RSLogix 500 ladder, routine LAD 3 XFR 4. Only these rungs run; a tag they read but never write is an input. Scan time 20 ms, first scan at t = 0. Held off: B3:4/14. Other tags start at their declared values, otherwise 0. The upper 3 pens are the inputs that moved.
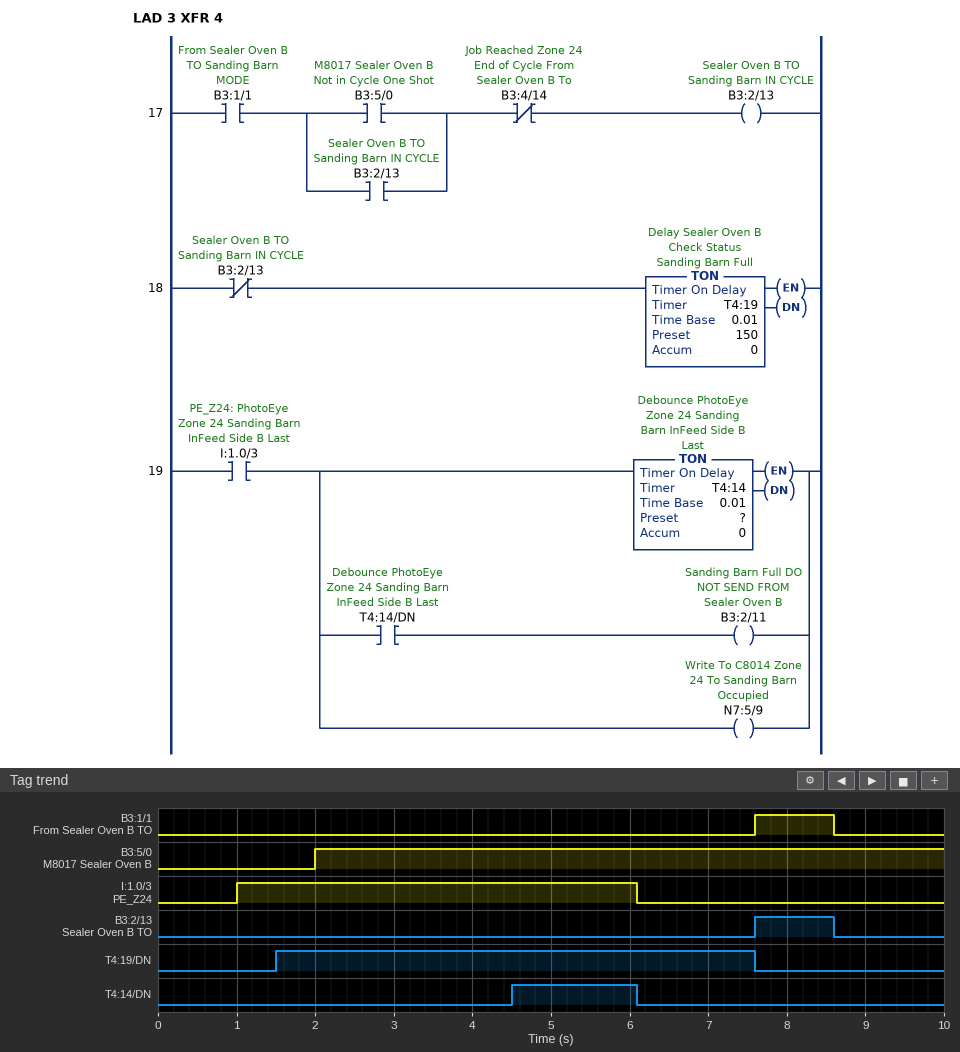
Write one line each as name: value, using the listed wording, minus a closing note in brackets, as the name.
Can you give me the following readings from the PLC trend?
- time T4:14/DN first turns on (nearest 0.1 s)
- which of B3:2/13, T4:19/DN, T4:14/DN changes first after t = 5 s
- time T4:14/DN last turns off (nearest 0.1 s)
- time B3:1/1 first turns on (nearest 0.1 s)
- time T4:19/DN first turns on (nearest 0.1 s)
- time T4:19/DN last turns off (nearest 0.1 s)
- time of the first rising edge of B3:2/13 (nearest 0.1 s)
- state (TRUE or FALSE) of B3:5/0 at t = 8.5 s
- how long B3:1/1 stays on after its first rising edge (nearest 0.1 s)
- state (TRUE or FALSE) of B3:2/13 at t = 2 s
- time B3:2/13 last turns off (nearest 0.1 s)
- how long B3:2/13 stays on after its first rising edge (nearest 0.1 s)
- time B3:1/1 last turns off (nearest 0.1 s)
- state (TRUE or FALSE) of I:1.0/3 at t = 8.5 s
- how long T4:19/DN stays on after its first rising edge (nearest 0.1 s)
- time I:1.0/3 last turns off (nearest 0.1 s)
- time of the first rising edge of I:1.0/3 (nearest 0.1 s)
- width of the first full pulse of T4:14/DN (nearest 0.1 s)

time T4:14/DN first turns on: 4.5 s
which of B3:2/13, T4:19/DN, T4:14/DN changes first after t = 5 s: T4:14/DN
time T4:14/DN last turns off: 6.1 s
time B3:1/1 first turns on: 7.6 s
time T4:19/DN first turns on: 1.5 s
time T4:19/DN last turns off: 7.6 s
time of the first rising edge of B3:2/13: 7.6 s
state (TRUE or FALSE) of B3:5/0 at t = 8.5 s: TRUE
how long B3:1/1 stays on after its first rising edge: 1.0 s
state (TRUE or FALSE) of B3:2/13 at t = 2 s: FALSE
time B3:2/13 last turns off: 8.6 s
how long B3:2/13 stays on after its first rising edge: 1.0 s
time B3:1/1 last turns off: 8.6 s
state (TRUE or FALSE) of I:1.0/3 at t = 8.5 s: FALSE
how long T4:19/DN stays on after its first rising edge: 6.1 s
time I:1.0/3 last turns off: 6.1 s
time of the first rising edge of I:1.0/3: 1.0 s
width of the first full pulse of T4:14/DN: 1.6 s
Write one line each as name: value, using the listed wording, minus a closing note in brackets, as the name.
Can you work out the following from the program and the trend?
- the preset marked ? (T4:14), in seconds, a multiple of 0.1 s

the preset marked ? (T4:14), in seconds, a multiple of 0.1 s: 3.5 s
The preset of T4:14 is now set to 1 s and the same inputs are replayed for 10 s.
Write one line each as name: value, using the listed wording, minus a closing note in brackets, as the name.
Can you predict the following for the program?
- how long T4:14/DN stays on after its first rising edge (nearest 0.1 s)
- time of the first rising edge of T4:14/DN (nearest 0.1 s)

how long T4:14/DN stays on after its first rising edge: 4.1 s
time of the first rising edge of T4:14/DN: 2.0 s
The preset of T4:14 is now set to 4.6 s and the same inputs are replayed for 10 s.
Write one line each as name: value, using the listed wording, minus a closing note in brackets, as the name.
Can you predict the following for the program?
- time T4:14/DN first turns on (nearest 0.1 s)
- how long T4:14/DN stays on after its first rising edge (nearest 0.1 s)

time T4:14/DN first turns on: 5.6 s
how long T4:14/DN stays on after its first rising edge: 0.5 s
